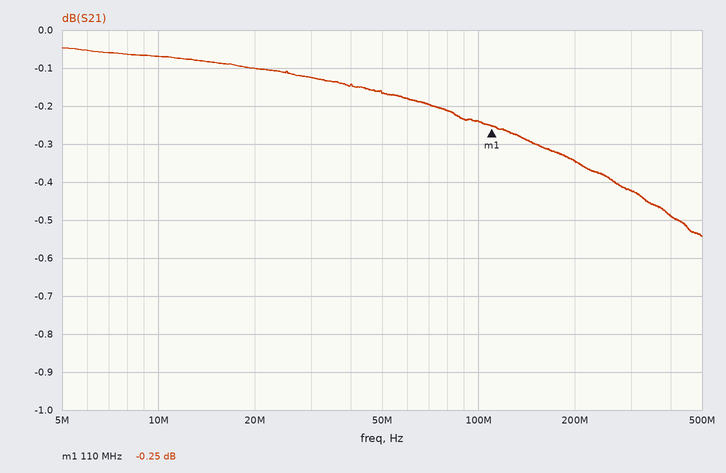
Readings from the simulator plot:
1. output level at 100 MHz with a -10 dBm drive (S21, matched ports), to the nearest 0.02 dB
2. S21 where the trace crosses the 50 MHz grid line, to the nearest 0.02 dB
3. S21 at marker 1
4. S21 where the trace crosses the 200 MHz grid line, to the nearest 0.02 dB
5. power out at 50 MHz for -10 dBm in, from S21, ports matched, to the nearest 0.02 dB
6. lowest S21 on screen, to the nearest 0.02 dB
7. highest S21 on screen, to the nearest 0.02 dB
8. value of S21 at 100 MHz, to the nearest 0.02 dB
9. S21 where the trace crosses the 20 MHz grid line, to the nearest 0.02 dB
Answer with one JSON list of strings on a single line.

["-10.24 dBm", "-0.16 dB", "-0.25 dB", "-0.34 dB", "-10.16 dBm", "-0.54 dB", "-0.04 dB", "-0.24 dB", "-0.10 dB"]
